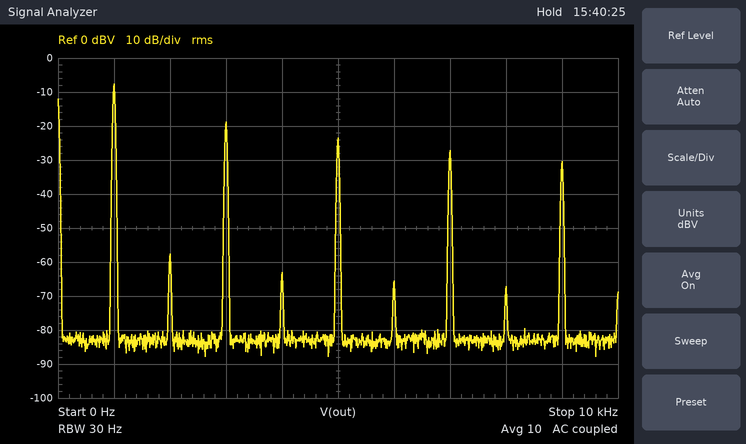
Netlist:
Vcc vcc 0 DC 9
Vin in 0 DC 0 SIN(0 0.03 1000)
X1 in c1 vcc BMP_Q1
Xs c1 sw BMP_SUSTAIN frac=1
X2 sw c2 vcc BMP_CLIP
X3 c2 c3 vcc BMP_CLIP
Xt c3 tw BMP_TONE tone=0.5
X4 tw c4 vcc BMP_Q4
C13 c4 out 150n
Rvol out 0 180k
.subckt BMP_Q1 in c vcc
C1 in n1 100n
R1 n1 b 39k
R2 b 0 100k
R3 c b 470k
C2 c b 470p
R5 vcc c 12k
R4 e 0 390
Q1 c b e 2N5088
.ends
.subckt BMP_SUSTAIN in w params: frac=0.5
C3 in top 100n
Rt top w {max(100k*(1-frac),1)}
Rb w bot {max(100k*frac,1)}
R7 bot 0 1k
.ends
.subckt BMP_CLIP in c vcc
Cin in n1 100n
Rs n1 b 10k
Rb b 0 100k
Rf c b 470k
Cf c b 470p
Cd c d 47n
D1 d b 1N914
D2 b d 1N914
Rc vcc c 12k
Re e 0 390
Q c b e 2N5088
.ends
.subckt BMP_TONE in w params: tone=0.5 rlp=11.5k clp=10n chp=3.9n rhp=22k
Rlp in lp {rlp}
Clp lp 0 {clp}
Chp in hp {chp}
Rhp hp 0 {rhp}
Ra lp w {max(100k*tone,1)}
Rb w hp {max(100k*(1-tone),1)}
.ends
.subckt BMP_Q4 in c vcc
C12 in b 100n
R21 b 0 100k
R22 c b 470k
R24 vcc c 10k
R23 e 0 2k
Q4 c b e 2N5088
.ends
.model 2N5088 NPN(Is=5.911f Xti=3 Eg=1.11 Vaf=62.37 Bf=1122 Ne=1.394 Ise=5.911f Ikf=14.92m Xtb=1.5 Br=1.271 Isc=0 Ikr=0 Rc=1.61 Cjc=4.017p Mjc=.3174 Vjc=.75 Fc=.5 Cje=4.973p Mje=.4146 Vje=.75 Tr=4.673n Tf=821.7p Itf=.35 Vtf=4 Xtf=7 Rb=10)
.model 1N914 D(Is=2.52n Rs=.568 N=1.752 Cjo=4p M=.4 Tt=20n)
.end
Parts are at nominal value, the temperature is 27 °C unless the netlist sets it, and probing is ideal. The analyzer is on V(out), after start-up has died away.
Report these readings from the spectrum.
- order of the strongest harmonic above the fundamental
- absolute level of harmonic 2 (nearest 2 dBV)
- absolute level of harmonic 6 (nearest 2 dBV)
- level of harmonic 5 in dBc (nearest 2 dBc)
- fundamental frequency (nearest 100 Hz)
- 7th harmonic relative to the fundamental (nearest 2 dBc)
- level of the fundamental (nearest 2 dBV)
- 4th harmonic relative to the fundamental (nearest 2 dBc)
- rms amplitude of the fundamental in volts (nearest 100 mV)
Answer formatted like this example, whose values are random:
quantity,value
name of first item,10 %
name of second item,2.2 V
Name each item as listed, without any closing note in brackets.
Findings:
quantity,value
order of the strongest harmonic above the fundamental,3
absolute level of harmonic 2,-58 dBV
absolute level of harmonic 6,-66 dBV
level of harmonic 5 in dBc,-16 dBc
fundamental frequency,1.0 kHz
7th harmonic relative to the fundamental,-20 dBc
level of the fundamental,-8 dBV
4th harmonic relative to the fundamental,-56 dBc
rms amplitude of the fundamental in volts,400 mV
